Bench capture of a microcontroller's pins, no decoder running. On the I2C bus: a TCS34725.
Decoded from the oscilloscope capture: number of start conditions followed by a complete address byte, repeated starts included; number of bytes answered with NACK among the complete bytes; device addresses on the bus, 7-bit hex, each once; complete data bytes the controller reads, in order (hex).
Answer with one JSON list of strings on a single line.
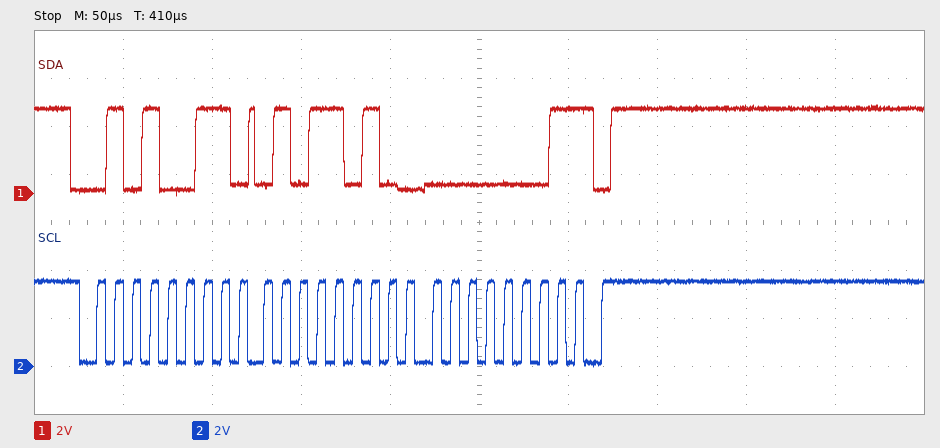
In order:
["1", "1", "0x29", "5A 01"]
